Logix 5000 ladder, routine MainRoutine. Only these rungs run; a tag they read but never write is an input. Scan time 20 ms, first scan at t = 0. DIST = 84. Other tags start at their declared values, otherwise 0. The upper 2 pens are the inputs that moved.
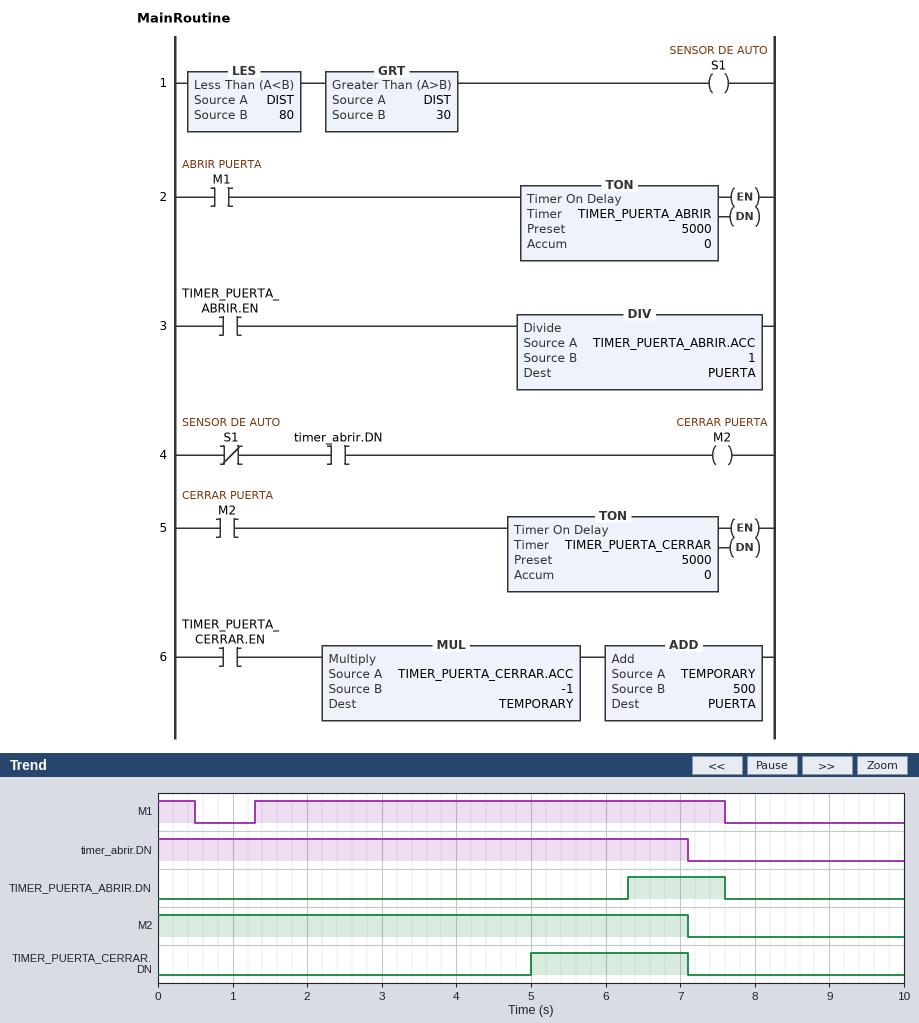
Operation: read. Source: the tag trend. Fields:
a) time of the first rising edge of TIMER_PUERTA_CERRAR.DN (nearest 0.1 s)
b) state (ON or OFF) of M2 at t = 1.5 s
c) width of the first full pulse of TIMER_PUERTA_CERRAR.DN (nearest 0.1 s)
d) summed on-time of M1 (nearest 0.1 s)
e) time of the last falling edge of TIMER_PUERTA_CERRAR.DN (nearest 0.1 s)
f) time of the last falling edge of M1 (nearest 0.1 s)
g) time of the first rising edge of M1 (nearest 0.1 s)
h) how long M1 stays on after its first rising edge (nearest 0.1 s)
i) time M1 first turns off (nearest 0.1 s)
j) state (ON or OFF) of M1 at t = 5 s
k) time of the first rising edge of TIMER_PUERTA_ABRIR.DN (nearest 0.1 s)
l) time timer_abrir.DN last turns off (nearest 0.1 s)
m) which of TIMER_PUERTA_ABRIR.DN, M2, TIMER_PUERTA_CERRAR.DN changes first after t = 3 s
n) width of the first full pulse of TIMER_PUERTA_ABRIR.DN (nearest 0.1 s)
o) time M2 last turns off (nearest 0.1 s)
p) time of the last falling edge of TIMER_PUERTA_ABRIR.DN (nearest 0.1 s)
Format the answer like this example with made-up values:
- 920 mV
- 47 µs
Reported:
- 5.0 s
- ON
- 2.1 s
- 6.8 s
- 7.1 s
- 7.6 s
- 1.3 s
- 6.3 s
- 0.5 s
- ON
- 6.3 s
- 7.1 s
- TIMER_PUERTA_CERRAR.DN
- 1.3 s
- 7.1 s
- 7.6 s
